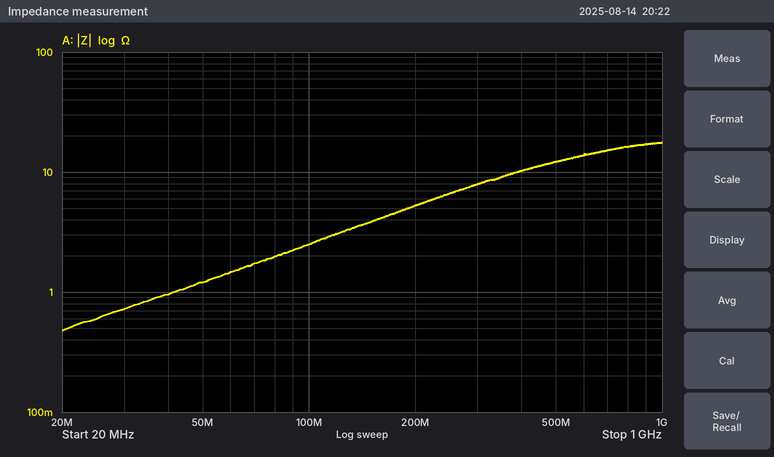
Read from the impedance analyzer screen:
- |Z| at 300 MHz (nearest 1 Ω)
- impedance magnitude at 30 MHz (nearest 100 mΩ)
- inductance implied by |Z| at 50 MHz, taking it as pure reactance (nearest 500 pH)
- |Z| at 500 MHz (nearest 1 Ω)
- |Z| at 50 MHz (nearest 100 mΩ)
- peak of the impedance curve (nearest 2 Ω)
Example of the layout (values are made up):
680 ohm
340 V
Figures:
8 Ω
700 mΩ
4.0 nH
12 Ω
1.2 Ω
18 Ω
